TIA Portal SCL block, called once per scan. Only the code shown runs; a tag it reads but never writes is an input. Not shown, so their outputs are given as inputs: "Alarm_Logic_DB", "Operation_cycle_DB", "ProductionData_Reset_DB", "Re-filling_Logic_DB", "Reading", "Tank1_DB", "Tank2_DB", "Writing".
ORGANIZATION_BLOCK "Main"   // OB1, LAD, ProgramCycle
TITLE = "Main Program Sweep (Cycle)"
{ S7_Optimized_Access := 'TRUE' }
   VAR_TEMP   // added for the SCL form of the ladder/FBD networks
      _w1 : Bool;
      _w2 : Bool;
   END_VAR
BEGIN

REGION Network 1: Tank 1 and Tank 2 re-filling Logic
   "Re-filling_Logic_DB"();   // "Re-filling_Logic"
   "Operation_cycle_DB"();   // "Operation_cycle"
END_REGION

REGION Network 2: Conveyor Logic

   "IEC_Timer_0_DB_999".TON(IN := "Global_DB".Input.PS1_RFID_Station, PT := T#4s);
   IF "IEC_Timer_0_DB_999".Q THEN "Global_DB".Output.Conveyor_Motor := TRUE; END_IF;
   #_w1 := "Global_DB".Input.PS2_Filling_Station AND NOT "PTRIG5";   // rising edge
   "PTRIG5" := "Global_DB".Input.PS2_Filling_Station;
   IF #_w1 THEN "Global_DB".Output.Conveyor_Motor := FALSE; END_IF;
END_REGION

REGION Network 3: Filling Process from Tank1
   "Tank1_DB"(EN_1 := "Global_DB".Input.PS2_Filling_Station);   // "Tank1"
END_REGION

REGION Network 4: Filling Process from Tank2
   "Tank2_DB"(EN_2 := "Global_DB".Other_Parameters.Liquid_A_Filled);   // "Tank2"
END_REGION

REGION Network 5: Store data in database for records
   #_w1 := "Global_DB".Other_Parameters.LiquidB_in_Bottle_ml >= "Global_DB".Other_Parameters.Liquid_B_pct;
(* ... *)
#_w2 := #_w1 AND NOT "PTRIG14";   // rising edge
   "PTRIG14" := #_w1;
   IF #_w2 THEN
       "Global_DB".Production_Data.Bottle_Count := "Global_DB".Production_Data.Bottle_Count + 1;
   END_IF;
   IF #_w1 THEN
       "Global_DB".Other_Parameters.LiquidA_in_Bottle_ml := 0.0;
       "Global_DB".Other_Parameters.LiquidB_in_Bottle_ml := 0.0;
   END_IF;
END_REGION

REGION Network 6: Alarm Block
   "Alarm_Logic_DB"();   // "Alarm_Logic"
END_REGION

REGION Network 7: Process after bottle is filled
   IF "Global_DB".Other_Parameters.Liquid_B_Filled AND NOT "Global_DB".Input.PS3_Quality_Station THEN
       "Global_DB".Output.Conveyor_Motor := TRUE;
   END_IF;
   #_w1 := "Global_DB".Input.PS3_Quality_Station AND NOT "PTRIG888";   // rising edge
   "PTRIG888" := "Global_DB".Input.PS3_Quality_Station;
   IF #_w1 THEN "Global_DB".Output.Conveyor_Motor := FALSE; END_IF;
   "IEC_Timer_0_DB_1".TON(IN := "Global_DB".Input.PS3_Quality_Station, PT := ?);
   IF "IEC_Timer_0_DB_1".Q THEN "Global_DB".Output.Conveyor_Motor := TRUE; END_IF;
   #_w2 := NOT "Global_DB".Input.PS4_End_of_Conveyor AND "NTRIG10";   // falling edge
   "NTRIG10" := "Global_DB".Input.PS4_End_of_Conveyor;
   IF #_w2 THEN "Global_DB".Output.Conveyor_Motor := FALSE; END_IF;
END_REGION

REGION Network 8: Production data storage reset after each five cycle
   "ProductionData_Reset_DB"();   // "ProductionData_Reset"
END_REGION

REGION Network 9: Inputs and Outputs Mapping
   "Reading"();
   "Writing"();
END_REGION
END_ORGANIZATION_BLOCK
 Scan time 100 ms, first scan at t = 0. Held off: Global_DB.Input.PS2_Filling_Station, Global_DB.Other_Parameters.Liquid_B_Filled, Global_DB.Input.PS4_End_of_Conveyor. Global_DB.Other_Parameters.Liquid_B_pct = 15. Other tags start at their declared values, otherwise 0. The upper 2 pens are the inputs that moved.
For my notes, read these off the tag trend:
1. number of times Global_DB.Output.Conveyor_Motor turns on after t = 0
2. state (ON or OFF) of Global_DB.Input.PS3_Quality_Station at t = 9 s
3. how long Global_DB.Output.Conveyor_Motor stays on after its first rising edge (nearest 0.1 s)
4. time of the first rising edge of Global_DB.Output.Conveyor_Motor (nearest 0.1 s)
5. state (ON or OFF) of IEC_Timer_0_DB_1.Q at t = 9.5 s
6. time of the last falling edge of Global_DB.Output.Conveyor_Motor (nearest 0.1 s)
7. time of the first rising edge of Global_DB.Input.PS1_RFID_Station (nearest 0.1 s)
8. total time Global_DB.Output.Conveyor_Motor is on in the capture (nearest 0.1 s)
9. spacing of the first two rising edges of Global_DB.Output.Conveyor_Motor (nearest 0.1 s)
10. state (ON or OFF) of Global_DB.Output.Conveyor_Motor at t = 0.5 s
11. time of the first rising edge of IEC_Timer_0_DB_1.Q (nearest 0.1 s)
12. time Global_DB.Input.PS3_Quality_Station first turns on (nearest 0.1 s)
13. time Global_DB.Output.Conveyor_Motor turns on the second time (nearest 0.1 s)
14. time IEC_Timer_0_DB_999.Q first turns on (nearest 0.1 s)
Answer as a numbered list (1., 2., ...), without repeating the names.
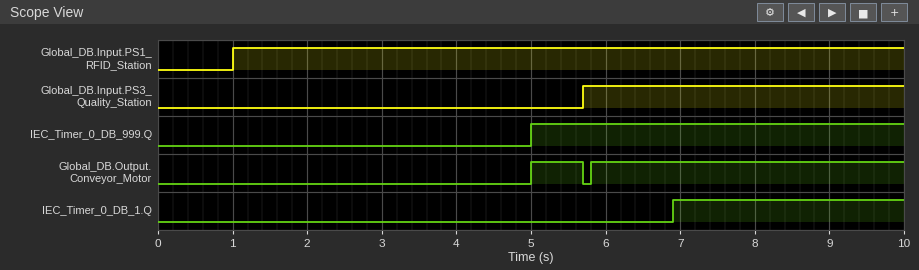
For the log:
1. 2
2. ON
3. 0.7 s
4. 5.0 s
5. ON
6. 5.7 s
7. 1.0 s
8. 4.9 s
9. 0.8 s
10. OFF
11. 6.9 s
12. 5.7 s
13. 5.8 s
14. 5.0 s
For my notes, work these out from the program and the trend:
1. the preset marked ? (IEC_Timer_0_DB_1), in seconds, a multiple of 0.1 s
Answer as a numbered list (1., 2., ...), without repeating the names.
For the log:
1. 1.2 s
